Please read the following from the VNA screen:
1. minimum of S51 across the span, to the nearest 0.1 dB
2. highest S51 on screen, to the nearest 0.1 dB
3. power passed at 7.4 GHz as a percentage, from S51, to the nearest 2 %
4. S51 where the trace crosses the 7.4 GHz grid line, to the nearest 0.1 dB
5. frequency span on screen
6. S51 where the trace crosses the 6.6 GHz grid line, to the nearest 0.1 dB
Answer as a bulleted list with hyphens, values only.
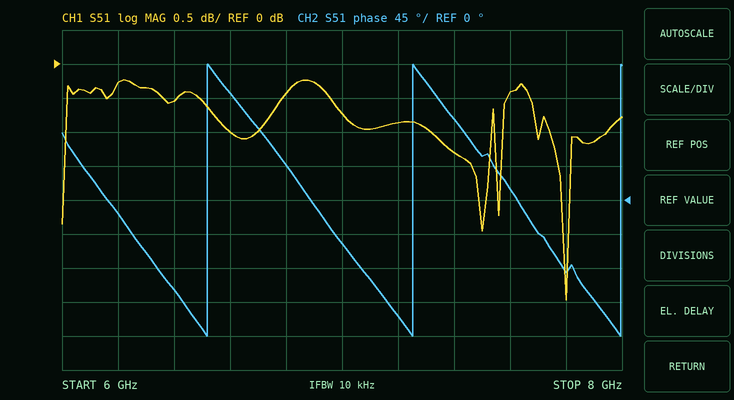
- -3.5 dB
- -0.2 dB
- 74 %
- -1.3 dB
- 2 GHz
- -1.0 dB
